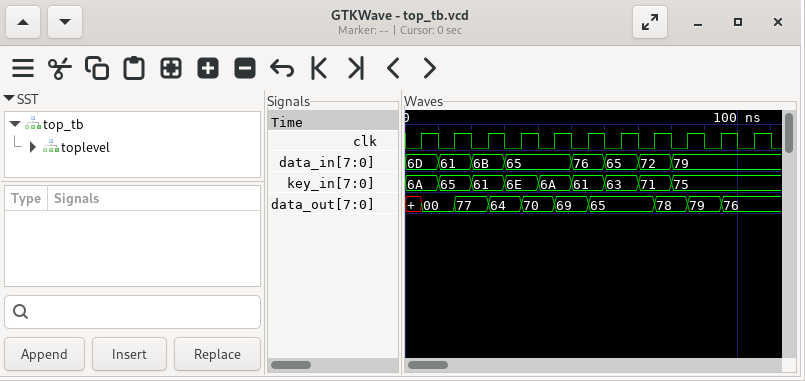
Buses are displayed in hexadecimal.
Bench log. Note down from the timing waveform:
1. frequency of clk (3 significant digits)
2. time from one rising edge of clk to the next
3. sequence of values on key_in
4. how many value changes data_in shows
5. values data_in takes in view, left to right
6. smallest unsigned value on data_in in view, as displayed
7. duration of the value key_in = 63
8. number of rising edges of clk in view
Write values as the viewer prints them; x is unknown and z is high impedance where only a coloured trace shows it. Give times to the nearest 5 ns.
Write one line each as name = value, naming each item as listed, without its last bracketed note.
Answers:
frequency of clk = 100 MHz
time from one rising edge of clk to the next = 10 ns
sequence of values on key_in = 6A, 65, 61, 6E, 6A, 61, 63, 71, 75
how many value changes data_in shows = 7
values data_in takes in view, left to right = 6D, 61, 6B, 65, 76, 65, 72, 79
smallest unsigned value on data_in in view, as displayed = 61
duration of the value key_in = 63 = 10 ns
number of rising edges of clk in view = 11
